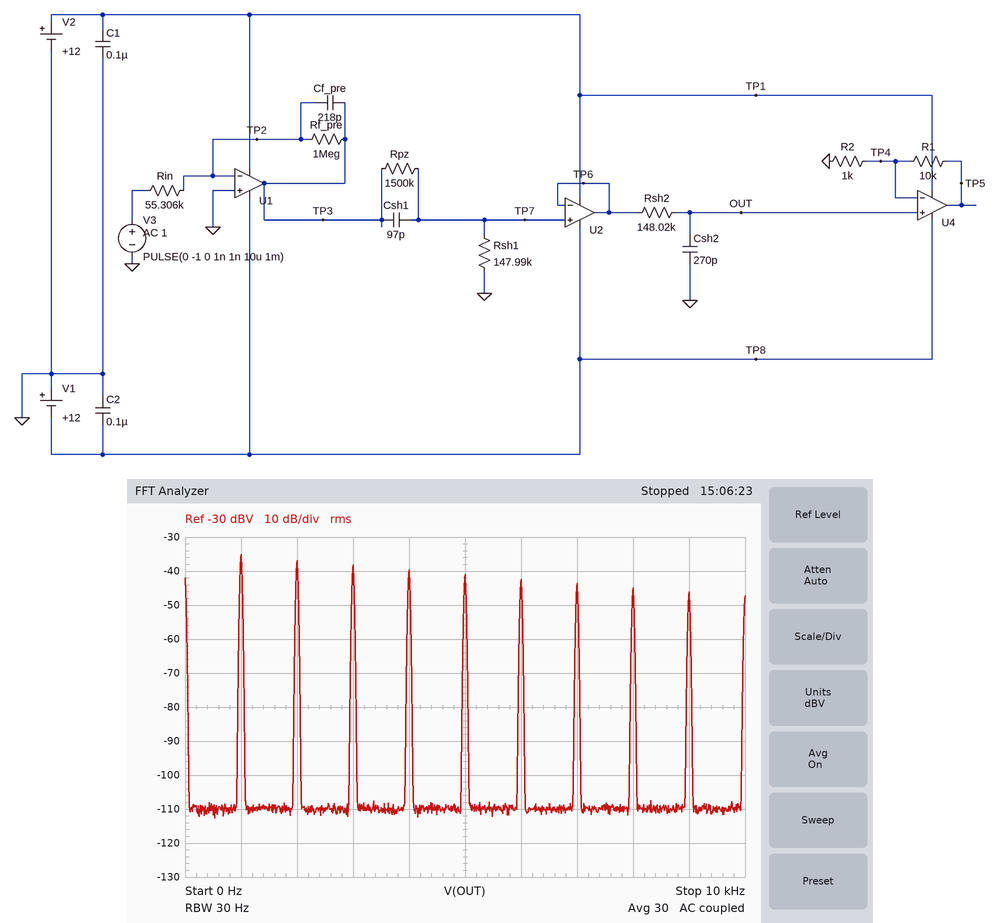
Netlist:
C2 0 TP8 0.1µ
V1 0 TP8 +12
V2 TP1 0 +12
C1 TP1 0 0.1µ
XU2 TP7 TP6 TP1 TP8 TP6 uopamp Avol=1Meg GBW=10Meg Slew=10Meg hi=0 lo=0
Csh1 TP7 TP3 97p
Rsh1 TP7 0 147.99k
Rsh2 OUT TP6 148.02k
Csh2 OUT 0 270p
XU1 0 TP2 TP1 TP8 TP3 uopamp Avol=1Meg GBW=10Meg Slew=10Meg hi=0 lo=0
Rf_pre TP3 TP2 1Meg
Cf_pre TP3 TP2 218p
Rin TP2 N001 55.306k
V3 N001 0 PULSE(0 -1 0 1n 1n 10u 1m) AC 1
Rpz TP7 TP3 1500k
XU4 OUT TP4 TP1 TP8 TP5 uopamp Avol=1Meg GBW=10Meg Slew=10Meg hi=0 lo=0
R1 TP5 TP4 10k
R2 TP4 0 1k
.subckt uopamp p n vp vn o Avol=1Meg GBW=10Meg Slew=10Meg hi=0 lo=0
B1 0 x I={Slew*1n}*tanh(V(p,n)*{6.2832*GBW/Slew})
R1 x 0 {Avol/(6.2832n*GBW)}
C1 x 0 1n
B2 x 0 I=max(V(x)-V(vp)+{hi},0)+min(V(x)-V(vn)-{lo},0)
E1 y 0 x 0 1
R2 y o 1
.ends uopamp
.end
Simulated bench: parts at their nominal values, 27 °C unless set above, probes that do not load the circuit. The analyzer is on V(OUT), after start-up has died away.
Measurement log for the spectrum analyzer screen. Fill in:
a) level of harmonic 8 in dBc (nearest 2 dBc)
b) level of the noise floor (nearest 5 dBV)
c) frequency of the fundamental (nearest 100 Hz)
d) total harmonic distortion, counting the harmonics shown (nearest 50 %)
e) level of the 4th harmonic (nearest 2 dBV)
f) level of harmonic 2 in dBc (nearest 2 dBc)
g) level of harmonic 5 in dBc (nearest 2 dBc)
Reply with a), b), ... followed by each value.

a) -10 dBc
b) -110 dBV
c) 1.0 kHz
d) 150 %
e) -40 dBV
f) -2 dBc
g) -6 dBc
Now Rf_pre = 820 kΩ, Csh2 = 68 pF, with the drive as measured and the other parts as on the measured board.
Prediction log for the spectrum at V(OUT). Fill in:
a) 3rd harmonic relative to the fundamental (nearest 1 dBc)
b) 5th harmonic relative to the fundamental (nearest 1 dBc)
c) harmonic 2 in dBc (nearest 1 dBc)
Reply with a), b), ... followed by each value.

a) -1 dBc
b) -2 dBc
c) -1 dBc
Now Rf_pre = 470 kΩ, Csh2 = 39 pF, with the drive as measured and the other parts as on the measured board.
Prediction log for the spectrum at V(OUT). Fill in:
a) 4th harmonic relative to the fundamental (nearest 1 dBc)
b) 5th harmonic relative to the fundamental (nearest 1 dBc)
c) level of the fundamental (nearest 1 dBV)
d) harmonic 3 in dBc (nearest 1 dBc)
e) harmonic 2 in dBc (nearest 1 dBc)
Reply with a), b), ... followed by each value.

a) 1 dBc
b) 1 dBc
c) -38 dBV
d) 1 dBc
e) 1 dBc
